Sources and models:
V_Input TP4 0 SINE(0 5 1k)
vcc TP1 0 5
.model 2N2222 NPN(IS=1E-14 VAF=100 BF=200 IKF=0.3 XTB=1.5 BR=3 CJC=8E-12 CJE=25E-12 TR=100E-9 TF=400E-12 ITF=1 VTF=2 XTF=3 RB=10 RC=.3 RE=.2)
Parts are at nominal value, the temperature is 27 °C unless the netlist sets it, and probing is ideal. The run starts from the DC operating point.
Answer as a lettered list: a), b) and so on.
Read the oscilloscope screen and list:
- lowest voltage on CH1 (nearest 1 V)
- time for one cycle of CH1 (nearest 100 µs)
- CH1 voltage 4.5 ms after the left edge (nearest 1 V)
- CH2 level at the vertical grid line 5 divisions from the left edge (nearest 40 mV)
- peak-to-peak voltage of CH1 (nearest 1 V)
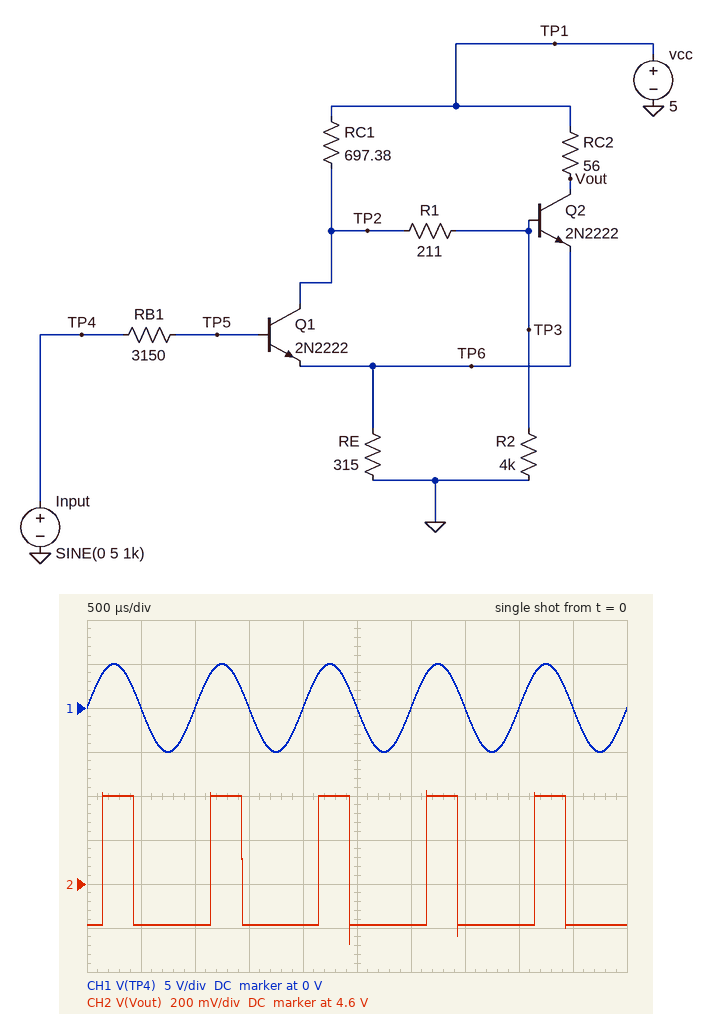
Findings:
a) -5 V
b) 1.0 ms
c) 0 V
d) 4.40 V
e) 10 V
